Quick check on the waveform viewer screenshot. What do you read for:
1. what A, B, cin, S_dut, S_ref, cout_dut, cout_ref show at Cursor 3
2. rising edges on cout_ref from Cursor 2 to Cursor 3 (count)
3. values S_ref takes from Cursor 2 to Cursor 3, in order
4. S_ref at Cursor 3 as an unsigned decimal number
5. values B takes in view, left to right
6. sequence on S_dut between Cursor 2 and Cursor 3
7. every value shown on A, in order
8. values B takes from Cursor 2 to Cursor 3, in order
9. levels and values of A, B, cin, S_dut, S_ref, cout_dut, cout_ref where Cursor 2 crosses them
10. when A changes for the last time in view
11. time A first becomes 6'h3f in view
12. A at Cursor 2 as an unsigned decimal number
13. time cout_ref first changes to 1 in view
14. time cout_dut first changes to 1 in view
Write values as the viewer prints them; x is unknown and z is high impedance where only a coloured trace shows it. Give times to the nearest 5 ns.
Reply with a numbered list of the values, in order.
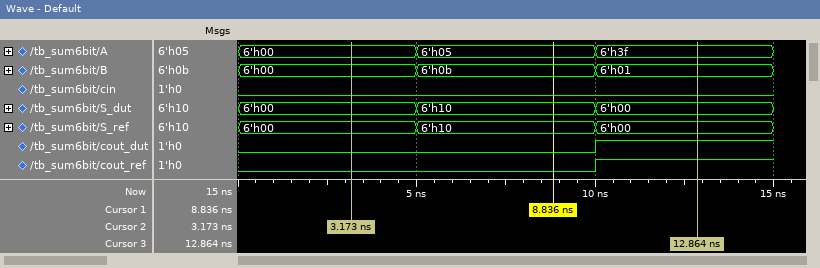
1. A=6'h3f, B=6'h01, cin=0, S_dut=6'h00, S_ref=6'h00, cout_dut=1, cout_ref=1
2. 1
3. 6'h00, 6'h10, 6'h00
4. 0
5. 6'h00, 6'h0b, 6'h01
6. 6'h00, 6'h10, 6'h00
7. 6'h00, 6'h05, 6'h3f
8. 6'h00, 6'h0b, 6'h01
9. A=6'h00, B=6'h00, cin=0, S_dut=6'h00, S_ref=6'h00, cout_dut=0, cout_ref=0
10. 10 ns
11. 10 ns
12. 0
13. 10 ns
14. 10 ns
